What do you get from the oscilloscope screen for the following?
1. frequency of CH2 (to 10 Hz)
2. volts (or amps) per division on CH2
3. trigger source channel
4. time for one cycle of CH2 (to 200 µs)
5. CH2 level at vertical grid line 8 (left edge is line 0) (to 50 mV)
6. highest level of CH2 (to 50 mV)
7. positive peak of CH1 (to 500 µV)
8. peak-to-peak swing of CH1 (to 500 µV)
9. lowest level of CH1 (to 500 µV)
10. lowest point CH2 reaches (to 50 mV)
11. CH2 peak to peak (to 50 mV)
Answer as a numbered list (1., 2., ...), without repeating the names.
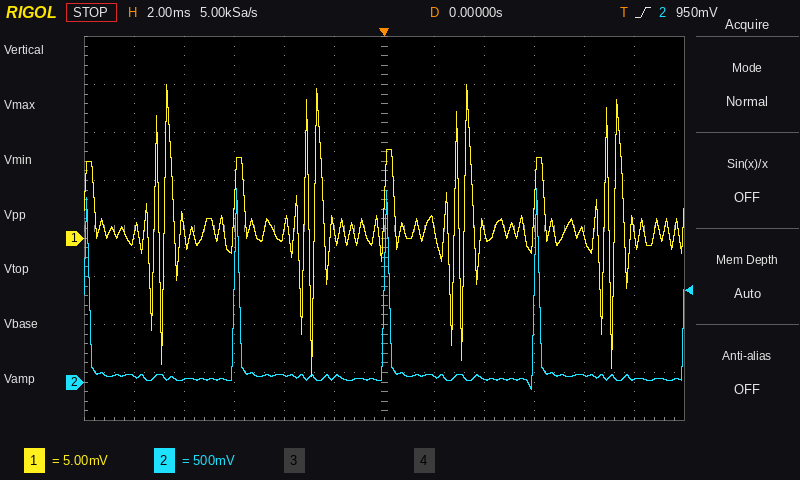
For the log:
1. 170 Hz
2. 500 mV
3. CH2
4. 6.0 ms
5. 50 mV
6. 2.00 V
7. 16.0 mV
8. 30.5 mV
9. -14.5 mV
10. -100 mV
11. 2.10 V
